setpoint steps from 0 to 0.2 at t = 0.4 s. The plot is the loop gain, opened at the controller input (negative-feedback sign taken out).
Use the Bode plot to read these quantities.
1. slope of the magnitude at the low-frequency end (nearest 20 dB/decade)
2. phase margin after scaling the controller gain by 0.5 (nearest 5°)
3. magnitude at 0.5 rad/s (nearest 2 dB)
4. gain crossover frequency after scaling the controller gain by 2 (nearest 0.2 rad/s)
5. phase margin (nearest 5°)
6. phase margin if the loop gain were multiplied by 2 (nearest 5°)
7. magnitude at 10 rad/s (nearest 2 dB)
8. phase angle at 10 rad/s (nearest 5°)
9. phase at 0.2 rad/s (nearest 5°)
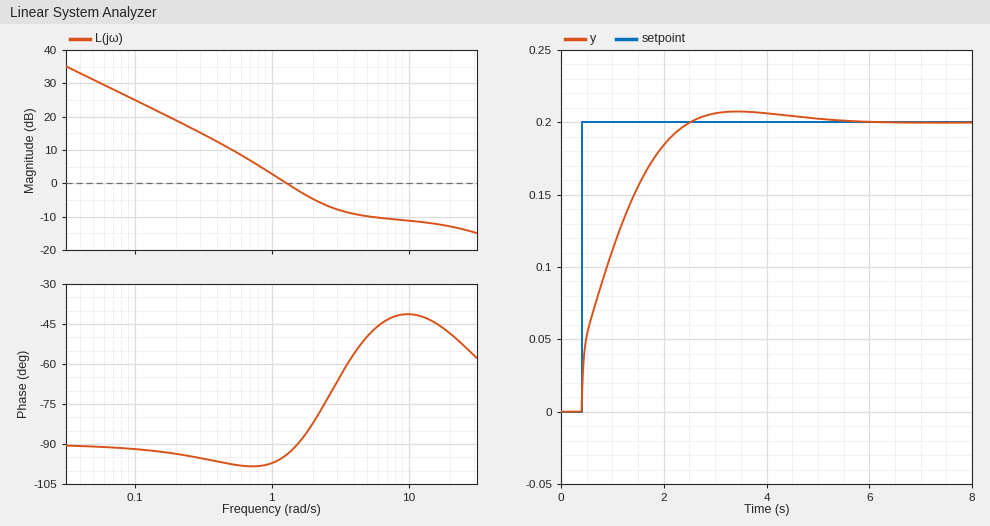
-20 dB/decade
80°
10 dB
2.4 rad/s
85°
105°
-12 dB
-40°
-95°
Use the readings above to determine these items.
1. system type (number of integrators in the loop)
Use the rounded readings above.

1
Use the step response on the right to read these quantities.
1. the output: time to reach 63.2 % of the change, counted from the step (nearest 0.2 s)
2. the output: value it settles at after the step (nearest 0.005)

0.8 s
0.200
